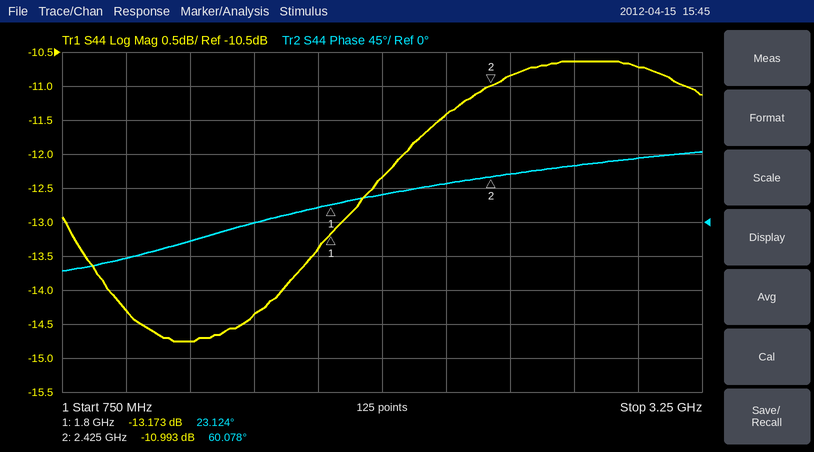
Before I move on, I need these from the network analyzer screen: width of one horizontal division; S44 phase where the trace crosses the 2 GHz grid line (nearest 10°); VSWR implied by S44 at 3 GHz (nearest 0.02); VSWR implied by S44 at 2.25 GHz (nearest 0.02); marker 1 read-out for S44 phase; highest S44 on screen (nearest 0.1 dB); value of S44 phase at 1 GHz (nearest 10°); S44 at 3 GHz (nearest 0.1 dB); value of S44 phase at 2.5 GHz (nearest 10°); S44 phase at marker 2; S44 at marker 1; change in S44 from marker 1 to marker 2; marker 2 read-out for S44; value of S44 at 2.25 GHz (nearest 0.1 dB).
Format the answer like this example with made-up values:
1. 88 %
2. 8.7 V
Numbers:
1. 250 MHz
2. 40°
3. 1.82
4. 1.74
5. 23.124°
6. -10.6 dB
7. -50°
8. -10.7 dB
9. 60°
10. 60.078°
11. -13.173 dB
12. 2.180 dB
13. -10.993 dB
14. -11.4 dB
